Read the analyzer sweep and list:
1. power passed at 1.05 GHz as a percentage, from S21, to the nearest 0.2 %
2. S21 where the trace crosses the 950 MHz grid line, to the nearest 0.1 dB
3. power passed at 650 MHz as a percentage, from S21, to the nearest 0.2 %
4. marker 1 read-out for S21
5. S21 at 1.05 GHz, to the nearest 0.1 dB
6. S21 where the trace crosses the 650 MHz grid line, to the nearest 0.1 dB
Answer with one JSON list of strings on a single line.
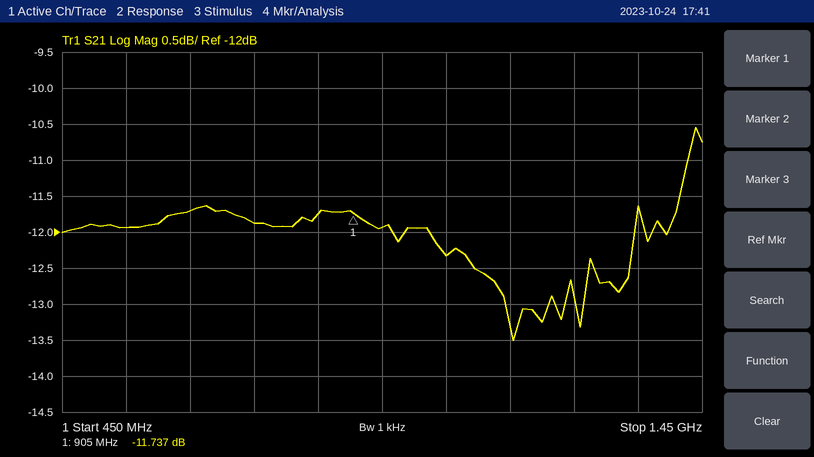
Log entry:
["5.8 %", "-11.9 dB", "6.8 %", "-11.737 dB", "-12.3 dB", "-11.7 dB"]
